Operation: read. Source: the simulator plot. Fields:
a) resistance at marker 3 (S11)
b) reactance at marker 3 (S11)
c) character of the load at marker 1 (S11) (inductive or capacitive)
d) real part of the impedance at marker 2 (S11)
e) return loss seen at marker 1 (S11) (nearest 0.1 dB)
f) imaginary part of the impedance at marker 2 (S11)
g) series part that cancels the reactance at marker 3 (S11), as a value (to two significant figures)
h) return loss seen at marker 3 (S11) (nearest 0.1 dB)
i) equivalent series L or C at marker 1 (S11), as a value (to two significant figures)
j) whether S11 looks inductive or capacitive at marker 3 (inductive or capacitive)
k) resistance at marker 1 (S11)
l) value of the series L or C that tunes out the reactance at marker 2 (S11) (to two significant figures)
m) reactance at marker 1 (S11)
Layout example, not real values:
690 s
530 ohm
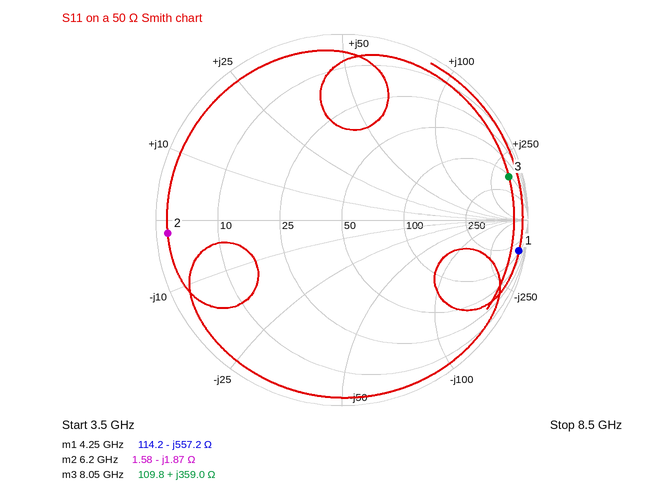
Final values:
109.8 Ω
+359.0 Ω
capacitive
1.58 Ω
0.3 dB
-1.87 Ω
55 fF
0.7 dB
67 fF
inductive
114.2 Ω
48 pH
-557.2 Ω
